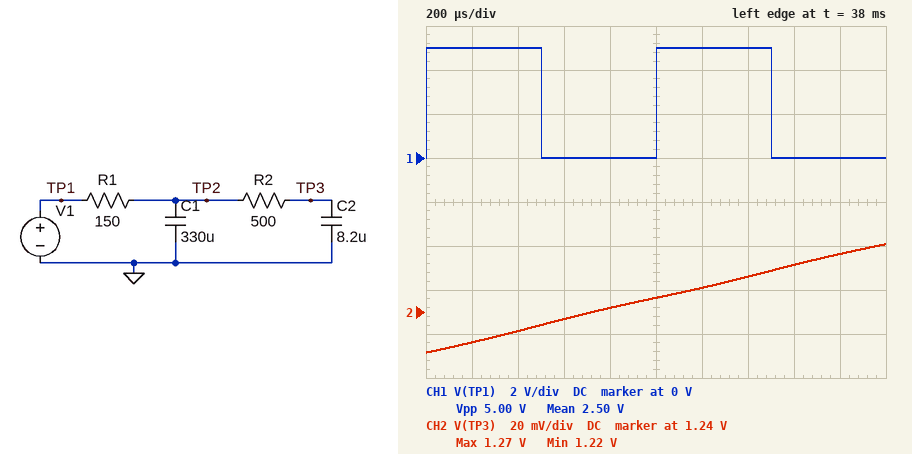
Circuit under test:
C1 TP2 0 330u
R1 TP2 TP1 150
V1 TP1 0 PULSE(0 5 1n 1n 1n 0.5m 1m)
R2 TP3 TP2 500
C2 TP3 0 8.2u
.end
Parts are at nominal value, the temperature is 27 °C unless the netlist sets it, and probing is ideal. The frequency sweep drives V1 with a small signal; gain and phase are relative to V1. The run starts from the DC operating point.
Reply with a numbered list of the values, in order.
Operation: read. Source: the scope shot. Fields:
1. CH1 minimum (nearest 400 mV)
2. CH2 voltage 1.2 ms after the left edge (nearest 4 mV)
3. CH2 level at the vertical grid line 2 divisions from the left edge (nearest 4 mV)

1. 0 V
2. 1.252 V
3. 1.232 V
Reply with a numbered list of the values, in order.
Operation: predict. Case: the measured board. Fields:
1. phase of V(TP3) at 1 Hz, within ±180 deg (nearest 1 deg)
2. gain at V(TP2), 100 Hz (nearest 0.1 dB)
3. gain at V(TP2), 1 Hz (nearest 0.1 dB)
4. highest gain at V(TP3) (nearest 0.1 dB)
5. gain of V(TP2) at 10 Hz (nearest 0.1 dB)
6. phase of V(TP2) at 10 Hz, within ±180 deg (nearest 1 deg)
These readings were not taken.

1. -19 deg
2. -29.9 dB
3. -0.4 dB
4. 0 dB
5. -10.5 dB
6. -72 deg
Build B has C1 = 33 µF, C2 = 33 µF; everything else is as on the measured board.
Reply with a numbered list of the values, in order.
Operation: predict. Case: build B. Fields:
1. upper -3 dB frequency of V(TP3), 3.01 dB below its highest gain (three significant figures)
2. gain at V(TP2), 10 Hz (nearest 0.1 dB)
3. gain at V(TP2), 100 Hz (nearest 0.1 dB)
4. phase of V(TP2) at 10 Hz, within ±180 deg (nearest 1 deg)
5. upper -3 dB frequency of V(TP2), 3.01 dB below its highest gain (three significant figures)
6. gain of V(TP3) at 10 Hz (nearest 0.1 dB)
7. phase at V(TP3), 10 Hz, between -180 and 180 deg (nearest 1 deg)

1. 6.81 Hz
2. -1.9 dB
3. -10.6 dB
4. -22 deg
5. 18.2 Hz
6. -5.1 dB
7. -68 deg
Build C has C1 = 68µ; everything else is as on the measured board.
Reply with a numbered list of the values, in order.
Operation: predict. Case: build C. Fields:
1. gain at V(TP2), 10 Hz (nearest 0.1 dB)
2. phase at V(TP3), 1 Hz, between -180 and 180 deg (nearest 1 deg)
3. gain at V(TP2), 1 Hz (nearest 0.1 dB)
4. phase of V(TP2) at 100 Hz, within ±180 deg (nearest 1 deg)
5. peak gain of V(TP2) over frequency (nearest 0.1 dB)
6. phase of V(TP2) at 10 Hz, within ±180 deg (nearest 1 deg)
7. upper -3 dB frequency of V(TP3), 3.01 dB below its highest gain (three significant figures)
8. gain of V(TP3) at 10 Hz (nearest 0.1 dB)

1. -1.9 dB
2. -6 deg
3. 0 dB
4. -79 deg
5. 0 dB
6. -35 deg
7. 12.3 Hz
8. -2.2 dB
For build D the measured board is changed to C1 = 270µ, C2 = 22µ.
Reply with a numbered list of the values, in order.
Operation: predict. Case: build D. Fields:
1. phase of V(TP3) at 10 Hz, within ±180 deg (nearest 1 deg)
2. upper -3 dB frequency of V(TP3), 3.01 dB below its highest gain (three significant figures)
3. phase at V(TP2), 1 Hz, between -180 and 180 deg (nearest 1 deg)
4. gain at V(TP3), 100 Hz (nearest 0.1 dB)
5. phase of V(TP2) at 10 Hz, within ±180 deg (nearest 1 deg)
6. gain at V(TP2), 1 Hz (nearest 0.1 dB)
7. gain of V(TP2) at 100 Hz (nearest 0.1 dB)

1. -102 deg
2. 3.39 Hz
3. -15 deg
4. -45.0 dB
5. -68 deg
6. -0.3 dB
7. -28.1 dB
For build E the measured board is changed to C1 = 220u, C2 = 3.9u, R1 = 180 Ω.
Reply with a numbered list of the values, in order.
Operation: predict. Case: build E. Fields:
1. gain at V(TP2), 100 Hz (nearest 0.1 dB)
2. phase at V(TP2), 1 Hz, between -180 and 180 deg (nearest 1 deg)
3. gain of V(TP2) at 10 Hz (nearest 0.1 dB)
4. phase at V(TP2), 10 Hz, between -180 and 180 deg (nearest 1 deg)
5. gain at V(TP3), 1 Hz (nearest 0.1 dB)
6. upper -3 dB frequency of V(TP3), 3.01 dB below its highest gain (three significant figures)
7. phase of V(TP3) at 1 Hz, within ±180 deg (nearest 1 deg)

1. -28.0 dB
2. -14 deg
3. -8.7 dB
4. -68 deg
5. -0.3 dB
6. 3.94 Hz
7. -15 deg
